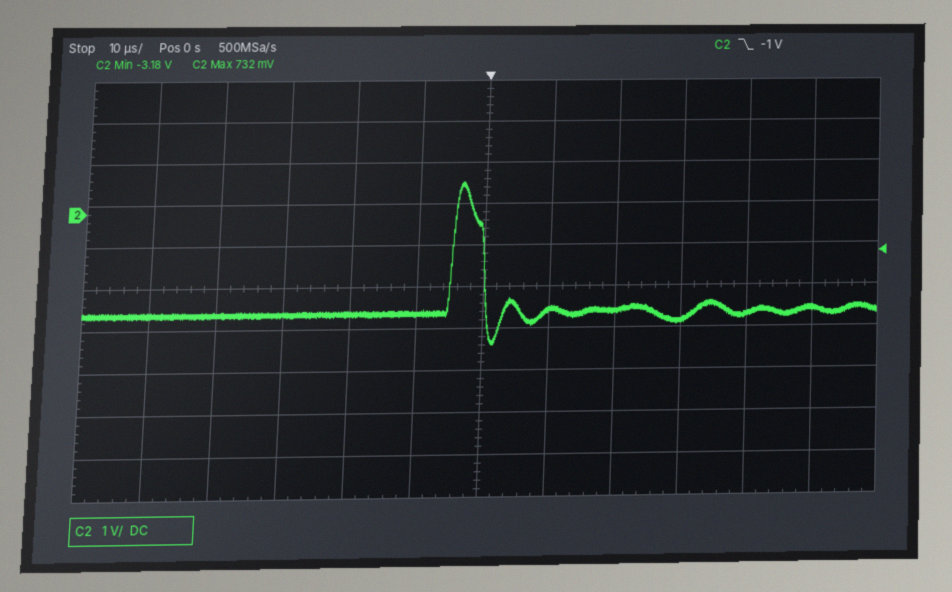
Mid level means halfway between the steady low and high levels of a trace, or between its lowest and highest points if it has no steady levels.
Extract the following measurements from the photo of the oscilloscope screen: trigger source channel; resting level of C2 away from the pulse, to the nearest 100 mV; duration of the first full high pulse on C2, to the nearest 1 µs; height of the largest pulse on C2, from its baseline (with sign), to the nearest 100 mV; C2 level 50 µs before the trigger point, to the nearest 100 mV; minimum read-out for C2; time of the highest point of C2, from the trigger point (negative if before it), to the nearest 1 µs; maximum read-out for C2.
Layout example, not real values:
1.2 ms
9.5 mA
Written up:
C2
-2.4 V
5 µs
+3.2 V
-2.4 V
-3.18 V
-3 µs
732 mV
